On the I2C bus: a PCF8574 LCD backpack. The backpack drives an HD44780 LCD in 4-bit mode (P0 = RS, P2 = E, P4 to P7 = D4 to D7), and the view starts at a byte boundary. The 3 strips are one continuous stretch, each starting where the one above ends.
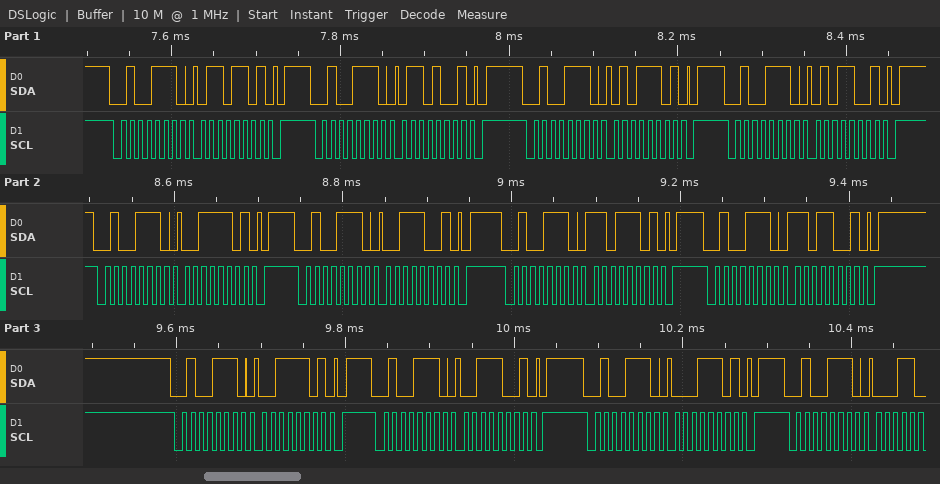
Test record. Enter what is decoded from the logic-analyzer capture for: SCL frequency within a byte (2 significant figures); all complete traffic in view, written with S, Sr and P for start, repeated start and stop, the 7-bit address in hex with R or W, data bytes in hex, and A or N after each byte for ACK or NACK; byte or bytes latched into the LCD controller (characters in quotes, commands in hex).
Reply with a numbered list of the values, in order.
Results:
1. 100 kHz
2. S 27W A 6D A P S 27W A 69 A P S 27W A 5D A P S 27W A 59 A P S 27W A 3D A P S 27W A 39 A P S 27W A DD A P S 27W A D9 A P S 27W A 3D A P S 27W A 39 A P S 27W A 1D A P S 27W A
3. 'e' '='
